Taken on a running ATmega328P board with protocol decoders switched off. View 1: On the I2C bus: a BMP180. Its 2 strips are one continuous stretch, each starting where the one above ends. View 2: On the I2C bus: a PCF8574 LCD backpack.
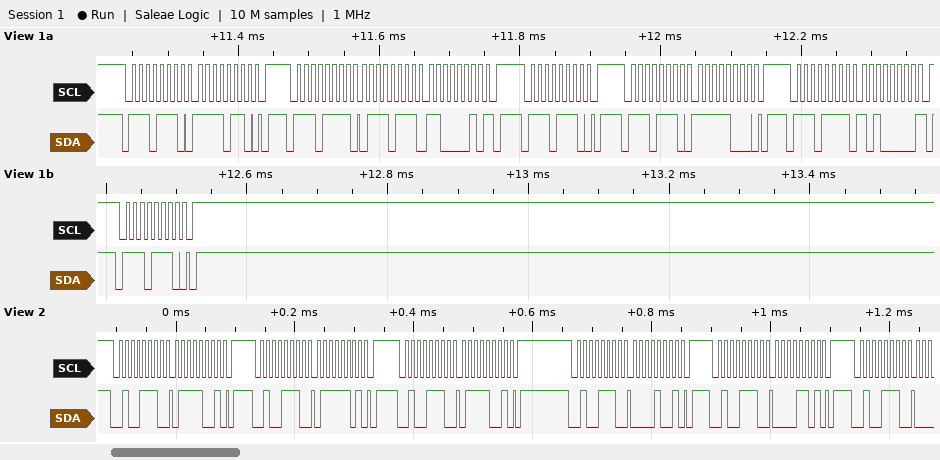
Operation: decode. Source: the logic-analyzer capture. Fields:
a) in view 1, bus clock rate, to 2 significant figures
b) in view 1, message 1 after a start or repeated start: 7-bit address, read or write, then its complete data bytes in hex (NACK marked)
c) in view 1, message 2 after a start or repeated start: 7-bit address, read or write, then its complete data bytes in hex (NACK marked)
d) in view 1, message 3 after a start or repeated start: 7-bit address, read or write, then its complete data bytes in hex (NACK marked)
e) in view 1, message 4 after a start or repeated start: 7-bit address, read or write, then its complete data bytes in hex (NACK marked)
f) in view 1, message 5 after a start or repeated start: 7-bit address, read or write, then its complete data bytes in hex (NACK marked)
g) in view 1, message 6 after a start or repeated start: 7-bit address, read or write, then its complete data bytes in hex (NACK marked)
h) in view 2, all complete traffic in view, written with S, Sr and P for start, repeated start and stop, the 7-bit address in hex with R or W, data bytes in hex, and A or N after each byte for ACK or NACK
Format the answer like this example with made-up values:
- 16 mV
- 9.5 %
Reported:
- 100 kHz
- 0x77 write: F6
- 0x77 read: 77 C2 NACK
- 0x77 write
- 0x77 write: F8
- 0x77 read: A0 NACK
- 0x77 write
- S 27W A 79 A P S 27W A 7D A P S 27W A 79 A P S 27W A 09 A P S 27W A 0D A P S 27W A
